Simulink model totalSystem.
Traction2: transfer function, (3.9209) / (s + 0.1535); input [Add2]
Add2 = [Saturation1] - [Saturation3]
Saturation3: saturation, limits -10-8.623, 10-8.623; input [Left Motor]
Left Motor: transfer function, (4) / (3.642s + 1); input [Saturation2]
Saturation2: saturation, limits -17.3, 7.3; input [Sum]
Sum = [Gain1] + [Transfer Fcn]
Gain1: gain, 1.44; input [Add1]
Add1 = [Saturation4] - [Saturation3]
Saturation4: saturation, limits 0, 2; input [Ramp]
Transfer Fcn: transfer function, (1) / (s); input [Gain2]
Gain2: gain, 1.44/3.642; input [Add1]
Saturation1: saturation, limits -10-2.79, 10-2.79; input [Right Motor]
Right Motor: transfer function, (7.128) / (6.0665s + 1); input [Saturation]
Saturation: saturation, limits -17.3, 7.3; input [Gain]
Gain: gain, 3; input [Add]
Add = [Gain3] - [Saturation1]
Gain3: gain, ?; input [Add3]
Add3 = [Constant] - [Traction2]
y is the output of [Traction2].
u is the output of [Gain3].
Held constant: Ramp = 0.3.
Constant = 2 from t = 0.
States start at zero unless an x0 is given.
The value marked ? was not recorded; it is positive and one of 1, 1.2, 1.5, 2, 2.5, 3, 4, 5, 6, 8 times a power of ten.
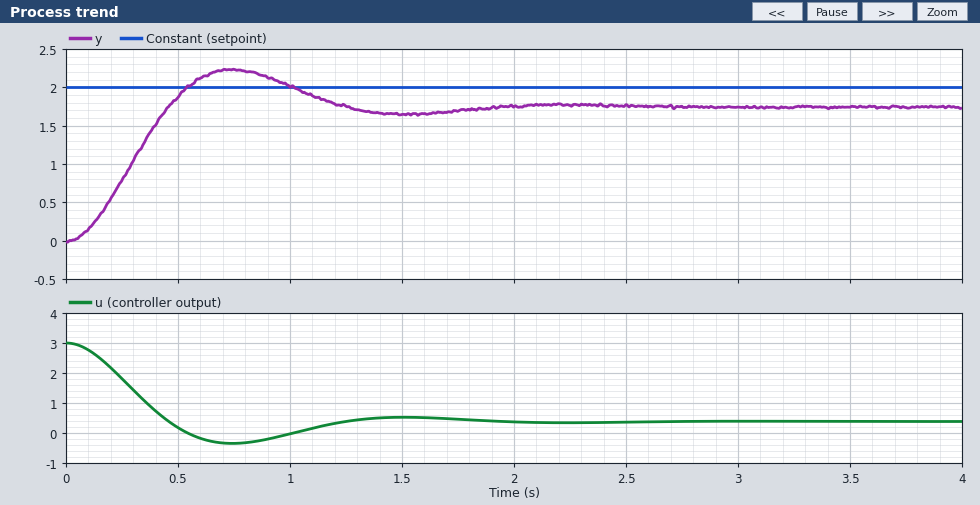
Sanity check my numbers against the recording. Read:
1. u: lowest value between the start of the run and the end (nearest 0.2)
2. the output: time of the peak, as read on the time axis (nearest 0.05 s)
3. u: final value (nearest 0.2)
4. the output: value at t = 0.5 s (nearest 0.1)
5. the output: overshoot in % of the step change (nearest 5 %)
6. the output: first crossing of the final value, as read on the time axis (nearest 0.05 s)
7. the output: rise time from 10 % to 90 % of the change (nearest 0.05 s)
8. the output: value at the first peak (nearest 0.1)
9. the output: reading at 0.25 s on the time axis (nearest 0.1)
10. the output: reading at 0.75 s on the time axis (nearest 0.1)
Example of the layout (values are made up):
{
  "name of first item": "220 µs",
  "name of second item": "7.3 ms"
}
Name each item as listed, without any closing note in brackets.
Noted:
{
  "u: lowest value between the start of the run and the end": "-0.4",
  "the output: time of the peak, as read on the time axis": "0.75 s",
  "u: final value": "0.4",
  "the output: value at t = 0.5 s": "1.9",
  "the output: overshoot in % of the step change": "30 %",
  "the output: first crossing of the final value, as read on the time axis": "0.45 s",
  "the output: rise time from 10 % to 90 % of the change": "0.30 s",
  "the output: value at the first peak": "2.2",
  "the output: reading at 0.25 s on the time axis": "0.8",
  "the output: reading at 0.75 s on the time axis": "2.2"
}
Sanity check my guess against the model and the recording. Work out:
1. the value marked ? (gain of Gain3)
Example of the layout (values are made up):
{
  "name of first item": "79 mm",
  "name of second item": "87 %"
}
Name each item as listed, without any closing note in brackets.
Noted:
{
  "the value marked ?": "1.5"
}
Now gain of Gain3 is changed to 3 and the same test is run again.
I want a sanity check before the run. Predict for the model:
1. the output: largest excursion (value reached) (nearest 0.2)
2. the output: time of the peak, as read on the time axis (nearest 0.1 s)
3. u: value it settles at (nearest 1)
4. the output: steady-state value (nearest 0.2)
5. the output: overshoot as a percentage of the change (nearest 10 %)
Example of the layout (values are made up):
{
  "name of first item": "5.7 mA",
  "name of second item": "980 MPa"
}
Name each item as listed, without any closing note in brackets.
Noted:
{
  "the output: largest excursion (value reached)": "2.6",
  "the output: time of the peak, as read on the time axis": "0.6 s",
  "u: value it settles at": "0",
  "the output: steady-state value": "1.8",
  "the output: overshoot as a percentage of the change": "40 %"
}
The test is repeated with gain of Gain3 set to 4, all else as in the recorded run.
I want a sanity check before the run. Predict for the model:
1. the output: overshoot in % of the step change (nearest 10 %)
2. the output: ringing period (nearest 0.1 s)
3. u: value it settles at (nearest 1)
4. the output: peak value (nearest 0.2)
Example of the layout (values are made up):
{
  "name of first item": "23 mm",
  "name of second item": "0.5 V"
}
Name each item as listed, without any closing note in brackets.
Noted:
{
  "the output: overshoot in % of the step change": "40 %",
  "the output: ringing period": "0.9 s",
  "u: value it settles at": "0",
  "the output: peak value": "2.6"
}
